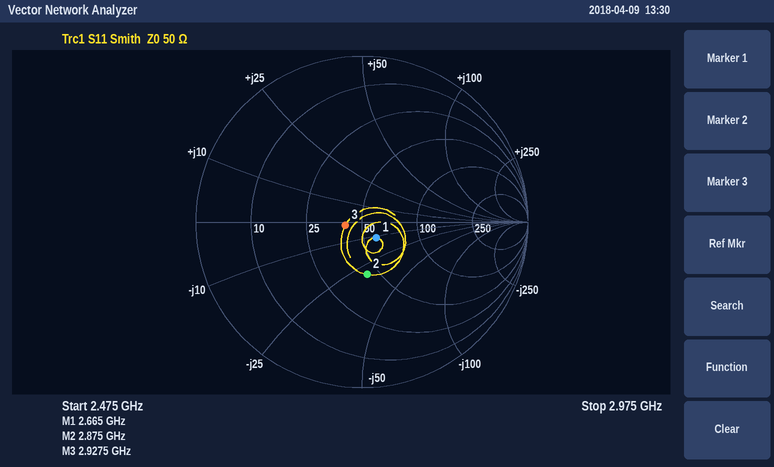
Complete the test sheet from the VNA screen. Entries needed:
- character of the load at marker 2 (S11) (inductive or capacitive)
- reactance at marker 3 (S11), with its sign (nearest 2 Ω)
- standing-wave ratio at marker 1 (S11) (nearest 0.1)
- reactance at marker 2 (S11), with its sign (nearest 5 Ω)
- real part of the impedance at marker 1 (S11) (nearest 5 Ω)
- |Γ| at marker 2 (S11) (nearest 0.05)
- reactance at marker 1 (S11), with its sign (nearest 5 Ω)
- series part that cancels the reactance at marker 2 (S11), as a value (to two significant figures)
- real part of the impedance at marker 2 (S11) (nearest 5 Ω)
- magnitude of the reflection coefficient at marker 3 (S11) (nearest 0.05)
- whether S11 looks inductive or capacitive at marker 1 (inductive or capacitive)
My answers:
capacitive
-2 Ω
1.3
-30 Ω
60 Ω
0.30
-10 Ω
1.7 nH
45 Ω
0.10
capacitive
